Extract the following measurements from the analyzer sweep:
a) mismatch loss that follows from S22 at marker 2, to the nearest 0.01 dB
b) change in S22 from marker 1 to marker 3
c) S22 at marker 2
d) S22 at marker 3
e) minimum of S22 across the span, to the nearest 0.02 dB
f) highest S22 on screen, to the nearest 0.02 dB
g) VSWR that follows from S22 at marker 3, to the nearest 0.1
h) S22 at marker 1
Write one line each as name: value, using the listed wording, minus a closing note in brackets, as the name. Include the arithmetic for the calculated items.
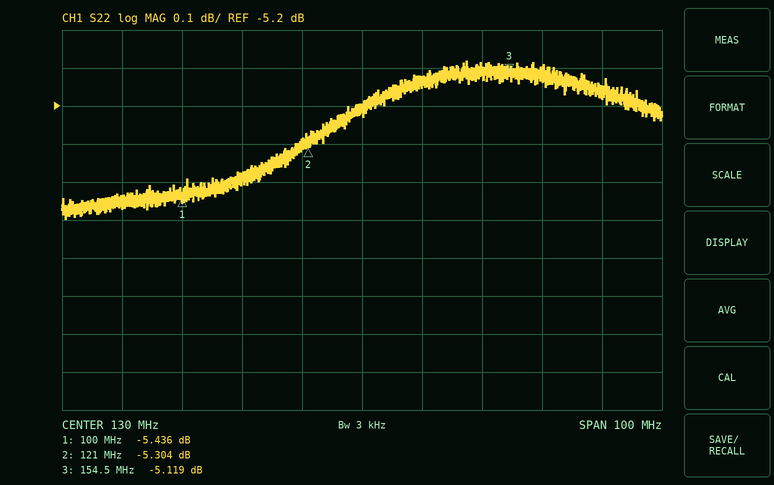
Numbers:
mismatch loss that follows from S22 at marker 2, to the nearest 0.01 dB: −10 log10(1 − 10^(-5.304/10)) ≈ 1.52 dB
change in S22 from marker 1 to marker 3: -5.119 − (-5.436) = 0.317 dB
S22 at marker 2: -5.304 dB
S22 at marker 3: -5.119 dB
minimum of S22 across the span, to the nearest 0.02 dB: -5.50 dB
highest S22 on screen, to the nearest 0.02 dB: -5.08 dB
VSWR that follows from S22 at marker 3, to the nearest 0.1: (1 + 0.5547)/(1 − 0.5547) ≈ 3.5
S22 at marker 1: -5.436 dB
